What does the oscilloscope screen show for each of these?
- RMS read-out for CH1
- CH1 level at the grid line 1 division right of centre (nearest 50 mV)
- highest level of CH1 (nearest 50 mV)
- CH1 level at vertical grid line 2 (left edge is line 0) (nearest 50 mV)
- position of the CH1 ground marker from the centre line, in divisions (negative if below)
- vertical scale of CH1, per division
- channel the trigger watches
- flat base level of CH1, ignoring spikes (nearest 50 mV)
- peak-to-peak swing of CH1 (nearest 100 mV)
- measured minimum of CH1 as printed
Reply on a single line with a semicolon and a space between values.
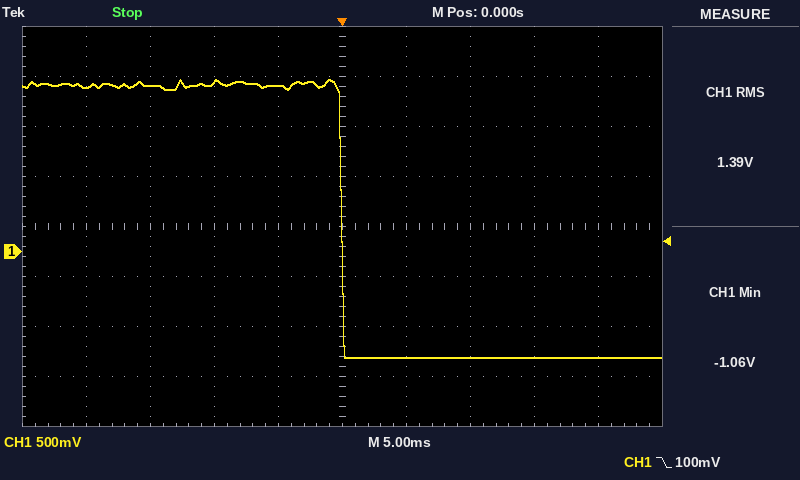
1.39 V; -1.05 V; 1.70 V; 1.65 V; -0.5 div; 500 mV; CH1; -1.05 V; 2.80 V; -1.06 V
